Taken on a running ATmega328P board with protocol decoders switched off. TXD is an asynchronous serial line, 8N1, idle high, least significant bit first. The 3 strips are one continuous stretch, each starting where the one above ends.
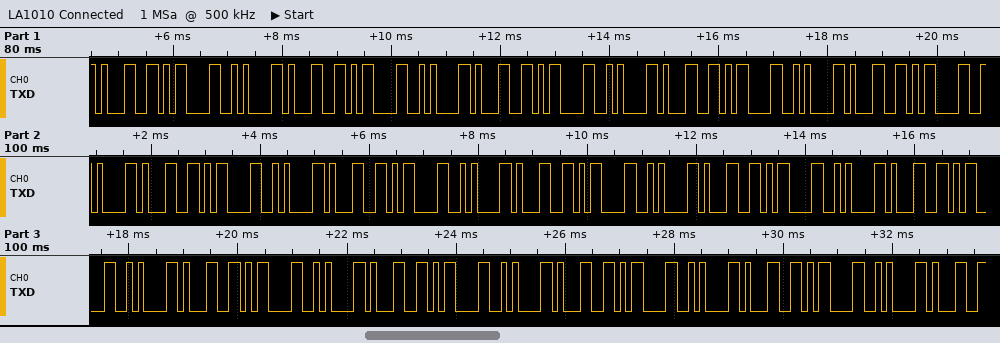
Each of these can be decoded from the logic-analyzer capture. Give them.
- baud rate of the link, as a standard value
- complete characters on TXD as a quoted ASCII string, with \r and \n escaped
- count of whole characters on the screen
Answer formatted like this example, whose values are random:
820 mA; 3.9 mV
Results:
9600 baud; "1\r\n1\r\n1\r\n1\r\n1\r\n1\r\n1\r\n1\r\n1\r\n1\r\n1\r\n1\r\n1\r\n1\r\n1"; 43
